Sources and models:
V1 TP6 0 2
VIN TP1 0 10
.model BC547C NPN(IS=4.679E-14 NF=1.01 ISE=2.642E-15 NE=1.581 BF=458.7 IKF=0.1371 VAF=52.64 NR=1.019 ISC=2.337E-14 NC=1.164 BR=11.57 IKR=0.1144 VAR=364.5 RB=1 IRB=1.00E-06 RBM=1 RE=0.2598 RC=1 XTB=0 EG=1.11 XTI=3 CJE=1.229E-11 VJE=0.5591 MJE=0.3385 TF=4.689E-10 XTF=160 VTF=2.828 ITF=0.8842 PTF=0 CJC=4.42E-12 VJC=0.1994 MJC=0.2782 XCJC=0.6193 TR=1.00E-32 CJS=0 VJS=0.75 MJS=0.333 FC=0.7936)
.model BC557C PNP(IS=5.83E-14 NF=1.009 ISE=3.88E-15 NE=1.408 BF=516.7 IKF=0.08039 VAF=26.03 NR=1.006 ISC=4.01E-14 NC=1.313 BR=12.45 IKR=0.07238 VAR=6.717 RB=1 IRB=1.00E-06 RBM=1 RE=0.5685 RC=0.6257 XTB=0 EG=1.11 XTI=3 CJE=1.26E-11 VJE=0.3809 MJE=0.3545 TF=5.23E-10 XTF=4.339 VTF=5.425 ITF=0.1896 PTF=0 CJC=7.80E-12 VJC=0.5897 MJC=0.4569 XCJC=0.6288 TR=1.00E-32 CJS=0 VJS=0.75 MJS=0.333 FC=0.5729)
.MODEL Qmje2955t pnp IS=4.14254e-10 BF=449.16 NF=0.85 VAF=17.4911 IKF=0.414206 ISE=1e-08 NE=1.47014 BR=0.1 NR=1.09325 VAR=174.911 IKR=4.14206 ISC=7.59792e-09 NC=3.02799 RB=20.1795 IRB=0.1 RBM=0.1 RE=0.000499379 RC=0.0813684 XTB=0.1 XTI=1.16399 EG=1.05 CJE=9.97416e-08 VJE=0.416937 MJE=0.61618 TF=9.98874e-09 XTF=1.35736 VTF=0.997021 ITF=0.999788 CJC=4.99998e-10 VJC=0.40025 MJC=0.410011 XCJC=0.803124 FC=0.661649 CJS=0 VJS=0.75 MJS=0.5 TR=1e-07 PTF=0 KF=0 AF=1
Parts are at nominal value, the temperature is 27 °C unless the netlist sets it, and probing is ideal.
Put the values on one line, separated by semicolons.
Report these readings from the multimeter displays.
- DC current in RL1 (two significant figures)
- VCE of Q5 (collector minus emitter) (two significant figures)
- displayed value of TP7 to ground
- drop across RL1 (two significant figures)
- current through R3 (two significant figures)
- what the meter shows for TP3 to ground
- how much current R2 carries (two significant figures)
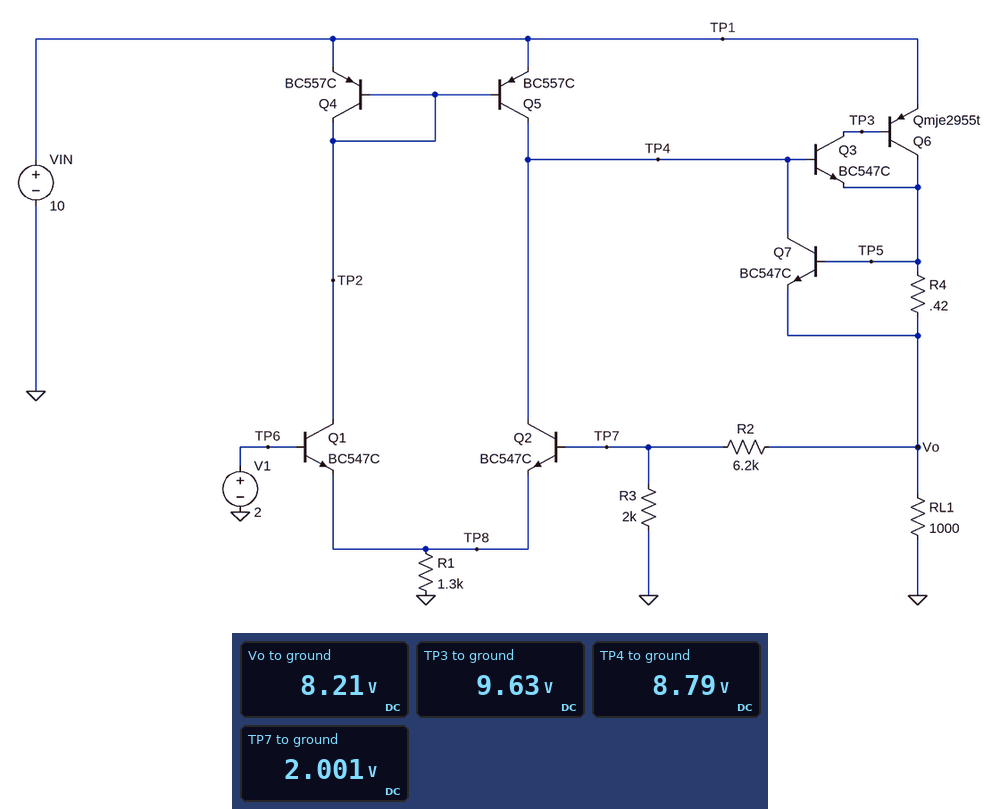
8.2 mA; -1.2 V; 2.001 V; 8.2 V; 1.0 mA; 9.63 V; 1.0 mA
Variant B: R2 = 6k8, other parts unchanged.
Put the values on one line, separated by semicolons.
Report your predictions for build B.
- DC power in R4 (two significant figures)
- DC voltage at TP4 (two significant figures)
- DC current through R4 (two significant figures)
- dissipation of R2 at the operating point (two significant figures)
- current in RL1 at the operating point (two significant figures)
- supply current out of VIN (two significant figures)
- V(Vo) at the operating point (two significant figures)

40 µW; 9.4 V; 9.8 mA; 6.8 mW; 8.8 mA; 11 mA; 8.8 V
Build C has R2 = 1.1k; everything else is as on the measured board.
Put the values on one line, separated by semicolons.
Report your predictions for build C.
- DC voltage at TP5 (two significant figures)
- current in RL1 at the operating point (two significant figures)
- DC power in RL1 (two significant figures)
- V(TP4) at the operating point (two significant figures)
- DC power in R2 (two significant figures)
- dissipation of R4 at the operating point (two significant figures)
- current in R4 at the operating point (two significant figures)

3.1 V; 3.1 mA; 9.7 mW; 3.7 V; 1.1 mW; 7.1 µW; 4.1 mA
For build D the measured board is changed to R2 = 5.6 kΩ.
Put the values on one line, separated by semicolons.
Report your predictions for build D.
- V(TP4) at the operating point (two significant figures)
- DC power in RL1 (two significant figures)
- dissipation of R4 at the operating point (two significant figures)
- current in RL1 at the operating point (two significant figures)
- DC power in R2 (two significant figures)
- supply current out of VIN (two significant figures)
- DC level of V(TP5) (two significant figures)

8.2 V; 58 mW; 31 µW; 7.6 mA; 5.6 mW; 9.7 mA; 7.6 V
